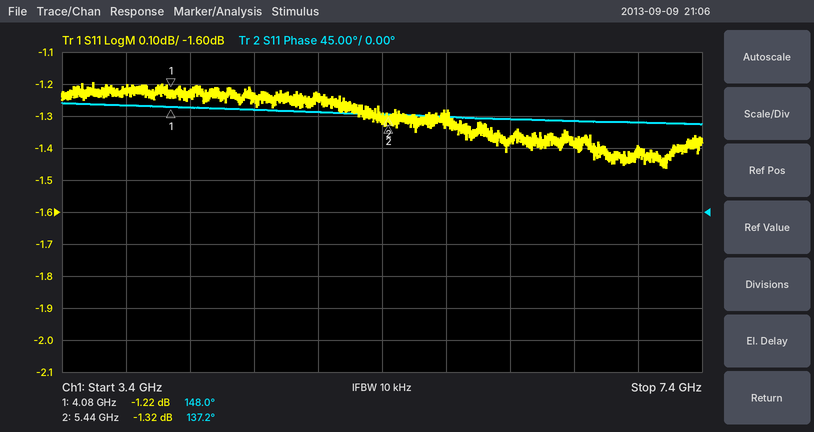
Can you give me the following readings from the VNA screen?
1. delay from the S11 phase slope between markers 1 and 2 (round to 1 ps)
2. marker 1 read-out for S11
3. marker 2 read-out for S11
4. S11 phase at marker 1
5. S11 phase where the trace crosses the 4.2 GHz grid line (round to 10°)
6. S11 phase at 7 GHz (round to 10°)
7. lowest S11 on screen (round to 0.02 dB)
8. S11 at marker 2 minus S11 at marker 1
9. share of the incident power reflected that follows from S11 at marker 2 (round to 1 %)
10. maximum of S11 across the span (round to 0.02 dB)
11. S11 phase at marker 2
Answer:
22 ps
-1.22 dB
-1.32 dB
148.0°
150°
130°
-1.46 dB
-0.10 dB
74 %
-1.20 dB
137.2°
